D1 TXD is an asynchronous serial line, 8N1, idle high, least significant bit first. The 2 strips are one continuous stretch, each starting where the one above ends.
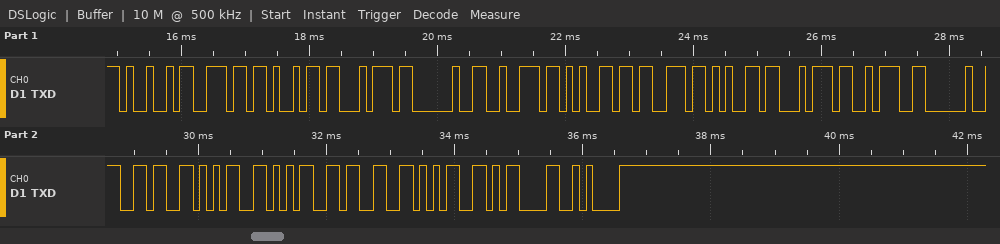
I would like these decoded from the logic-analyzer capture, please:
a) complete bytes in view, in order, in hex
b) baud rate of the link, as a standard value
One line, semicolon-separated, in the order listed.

0x49 0x6E 0x69 0x74 0x20 0x72 0x65 0x73 0x65 0x74 0x3A 0x20 0x36 0x35 0x35 0x33 0x35 0x0D 0x0A; 9600 baud
